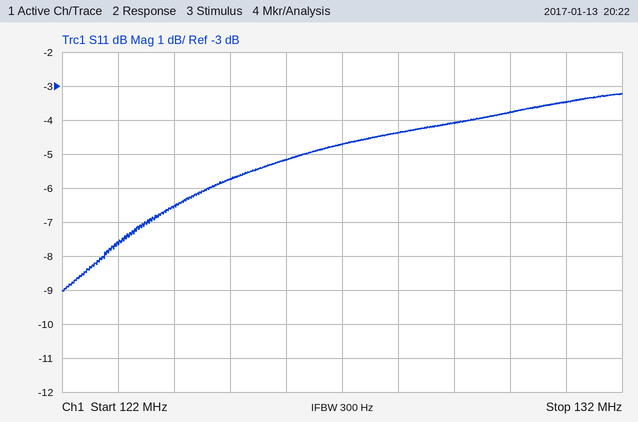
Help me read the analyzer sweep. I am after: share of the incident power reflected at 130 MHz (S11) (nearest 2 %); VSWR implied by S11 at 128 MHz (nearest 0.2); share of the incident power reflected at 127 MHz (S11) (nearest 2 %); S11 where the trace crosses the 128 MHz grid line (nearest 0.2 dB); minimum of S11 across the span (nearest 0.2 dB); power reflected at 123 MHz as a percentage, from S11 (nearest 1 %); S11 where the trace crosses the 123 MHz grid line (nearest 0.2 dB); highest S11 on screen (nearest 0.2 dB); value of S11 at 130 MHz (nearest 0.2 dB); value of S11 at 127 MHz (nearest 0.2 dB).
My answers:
42 %
4.0
34 %
-4.4 dB
-9.0 dB
17 %
-7.6 dB
-3.2 dB
-3.8 dB
-4.8 dB
